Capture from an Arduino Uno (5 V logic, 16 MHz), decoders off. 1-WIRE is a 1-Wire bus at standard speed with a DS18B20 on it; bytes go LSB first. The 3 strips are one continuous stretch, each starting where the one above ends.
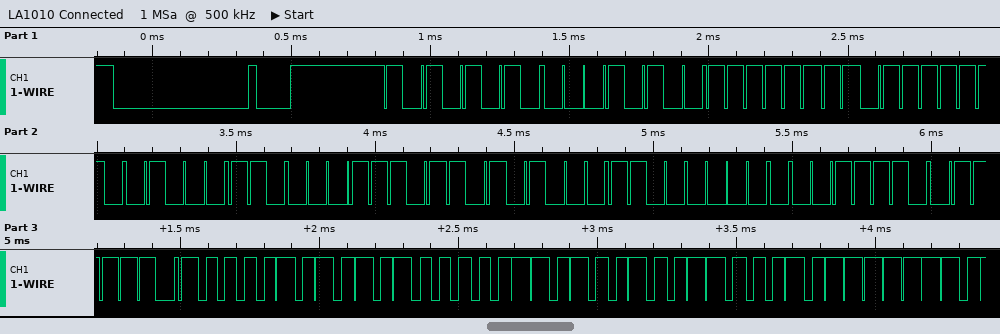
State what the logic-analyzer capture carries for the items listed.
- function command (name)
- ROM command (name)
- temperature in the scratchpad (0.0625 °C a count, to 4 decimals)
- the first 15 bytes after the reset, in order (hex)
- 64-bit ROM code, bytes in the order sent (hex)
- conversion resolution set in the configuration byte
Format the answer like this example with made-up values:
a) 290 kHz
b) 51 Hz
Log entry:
a) Read Scratchpad
b) Match ROM
c) 85.0000 °C
d) 55 28 FF 7E 62 B8 15 03 78 BE 50 05 4B 46 7F
e) 28 FF 7E 62 B8 15 03 78
f) 12 bits
